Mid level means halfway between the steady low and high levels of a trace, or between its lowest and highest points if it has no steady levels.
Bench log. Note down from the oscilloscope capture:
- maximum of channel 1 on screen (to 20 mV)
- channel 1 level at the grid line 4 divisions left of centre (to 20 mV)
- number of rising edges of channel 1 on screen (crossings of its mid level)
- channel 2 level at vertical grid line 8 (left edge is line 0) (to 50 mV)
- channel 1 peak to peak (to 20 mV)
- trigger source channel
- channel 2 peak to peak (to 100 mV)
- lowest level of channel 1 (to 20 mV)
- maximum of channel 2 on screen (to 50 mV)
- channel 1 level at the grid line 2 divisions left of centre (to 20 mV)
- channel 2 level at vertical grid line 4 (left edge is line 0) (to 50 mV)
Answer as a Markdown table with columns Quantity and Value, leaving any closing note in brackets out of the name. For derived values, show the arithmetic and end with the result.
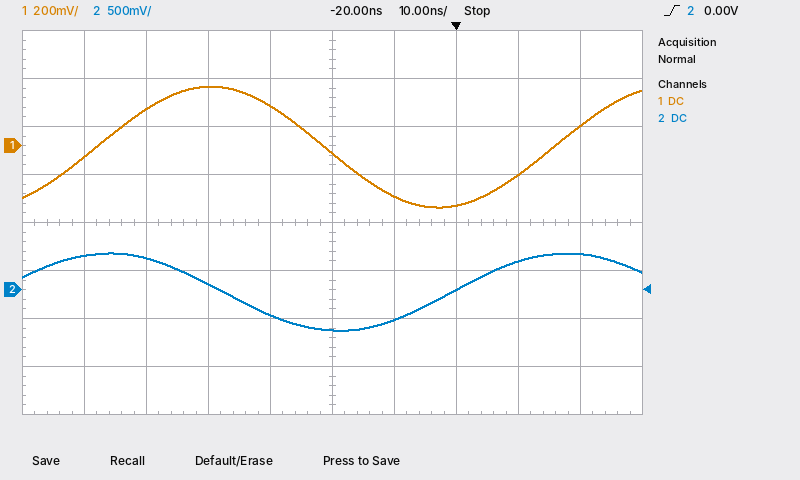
| Quantity | Value |
|---|---|
| maximum of channel 1 on screen | 240 mV |
| channel 1 level at the grid line 4 divisions left of centre | -40 mV |
| number of rising edges of channel 1 on screen | 2 |
| channel 2 level at vertical grid line 8 (left edge is line 0) | 300 mV |
| channel 1 peak to peak | 240 mV − (-260 mV) = 500 mV |
| trigger source channel | channel 2 |
| channel 2 peak to peak | 800 mV |
| lowest level of channel 1 | -260 mV |
| maximum of channel 2 on screen | 400 mV |
| channel 1 level at the grid line 2 divisions left of centre | 240 mV |
| channel 2 level at vertical grid line 4 (left edge is line 0) | -250 mV |
